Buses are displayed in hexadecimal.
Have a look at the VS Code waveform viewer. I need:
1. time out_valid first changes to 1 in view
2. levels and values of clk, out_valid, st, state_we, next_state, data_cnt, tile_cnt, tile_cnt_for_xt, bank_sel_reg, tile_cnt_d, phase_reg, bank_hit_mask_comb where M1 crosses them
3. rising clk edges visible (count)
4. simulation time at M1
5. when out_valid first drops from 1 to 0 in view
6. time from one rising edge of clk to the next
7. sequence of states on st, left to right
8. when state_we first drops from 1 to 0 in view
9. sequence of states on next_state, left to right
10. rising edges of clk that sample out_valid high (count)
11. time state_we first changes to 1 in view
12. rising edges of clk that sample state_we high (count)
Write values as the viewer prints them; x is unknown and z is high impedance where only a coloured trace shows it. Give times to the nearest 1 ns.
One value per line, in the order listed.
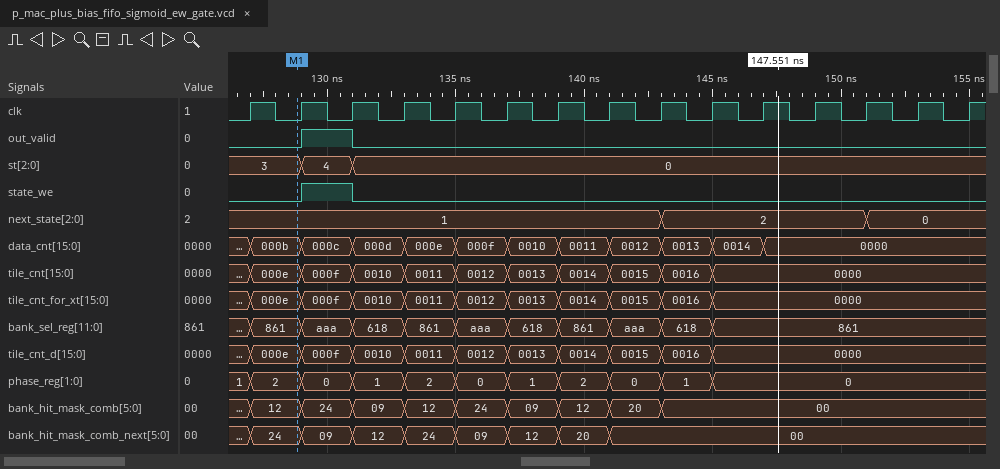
129 ns
clk=0, out_valid=0, st=3, state_we=0, next_state=1, data_cnt=000b, tile_cnt=000e, tile_cnt_for_xt=000e, bank_sel_reg=861, tile_cnt_d=000e, phase_reg=2, bank_hit_mask_comb=12
15
129 ns
131 ns
2 ns
3, 4, 0
131 ns
1, 2, 0
1
129 ns
1
